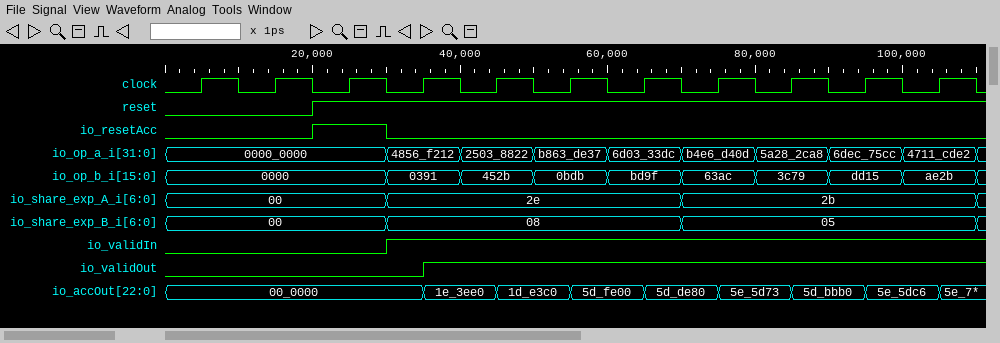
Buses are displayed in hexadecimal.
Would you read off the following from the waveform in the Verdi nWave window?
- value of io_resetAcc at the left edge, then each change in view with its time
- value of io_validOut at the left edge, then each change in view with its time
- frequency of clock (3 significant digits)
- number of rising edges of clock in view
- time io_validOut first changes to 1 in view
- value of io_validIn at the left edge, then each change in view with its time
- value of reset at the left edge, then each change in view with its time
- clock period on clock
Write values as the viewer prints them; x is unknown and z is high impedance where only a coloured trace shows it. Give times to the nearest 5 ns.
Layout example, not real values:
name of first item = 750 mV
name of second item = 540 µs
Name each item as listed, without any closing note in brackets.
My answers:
value of io_resetAcc at the left edge, then each change in view with its time = 0, 1 at 20 ns, 0 at 30 ns
value of io_validOut at the left edge, then each change in view with its time = 0, 1 at 35 ns
frequency of clock = 100 MHz
number of rising edges of clock in view = 11
time io_validOut first changes to 1 in view = 35 ns
value of io_validIn at the left edge, then each change in view with its time = 0, 1 at 30 ns
value of reset at the left edge, then each change in view with its time = 0, 1 at 20 ns
clock period on clock = 10 ns
